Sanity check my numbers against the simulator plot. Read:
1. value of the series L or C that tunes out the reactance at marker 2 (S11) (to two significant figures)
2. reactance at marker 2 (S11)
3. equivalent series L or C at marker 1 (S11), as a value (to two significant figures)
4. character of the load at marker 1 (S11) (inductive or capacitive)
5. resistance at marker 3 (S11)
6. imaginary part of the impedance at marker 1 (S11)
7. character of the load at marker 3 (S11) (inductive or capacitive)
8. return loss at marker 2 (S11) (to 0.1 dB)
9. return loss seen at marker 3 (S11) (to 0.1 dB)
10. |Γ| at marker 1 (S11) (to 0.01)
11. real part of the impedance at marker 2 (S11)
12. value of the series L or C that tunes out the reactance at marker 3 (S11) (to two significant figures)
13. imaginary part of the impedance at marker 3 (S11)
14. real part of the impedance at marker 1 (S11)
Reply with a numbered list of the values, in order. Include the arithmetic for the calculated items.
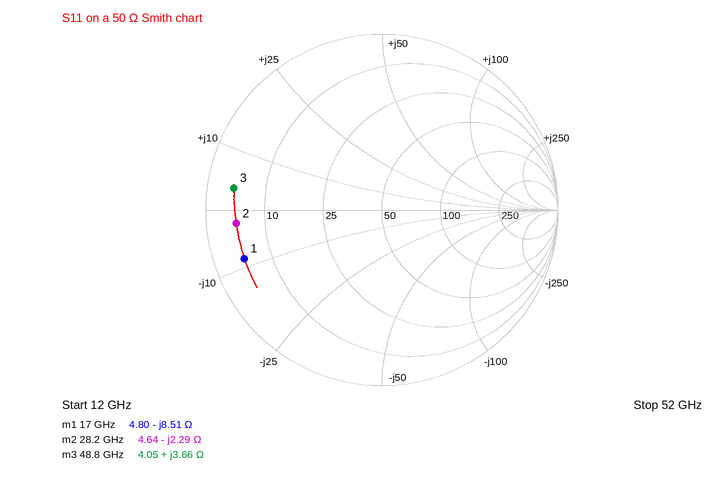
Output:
1. L = 2.29 Ω/(2π × 28.2 GHz) ≈ 13 pH
2. -2.29 Ω
3. C = 1/(2π × 17 GHz × 8.51 Ω) ≈ 1.1 pF
4. capacitive
5. 4.05 Ω
6. -8.51 Ω
7. inductive
8. 1.6 dB
9. 1.4 dB
10. 0.83
11. 4.64 Ω
12. C = 1/(2π × 48.8 GHz × 3.66 Ω) ≈ 891 fF, so 890 fF to two significant figures
13. +3.66 Ω
14. 4.80 Ω
